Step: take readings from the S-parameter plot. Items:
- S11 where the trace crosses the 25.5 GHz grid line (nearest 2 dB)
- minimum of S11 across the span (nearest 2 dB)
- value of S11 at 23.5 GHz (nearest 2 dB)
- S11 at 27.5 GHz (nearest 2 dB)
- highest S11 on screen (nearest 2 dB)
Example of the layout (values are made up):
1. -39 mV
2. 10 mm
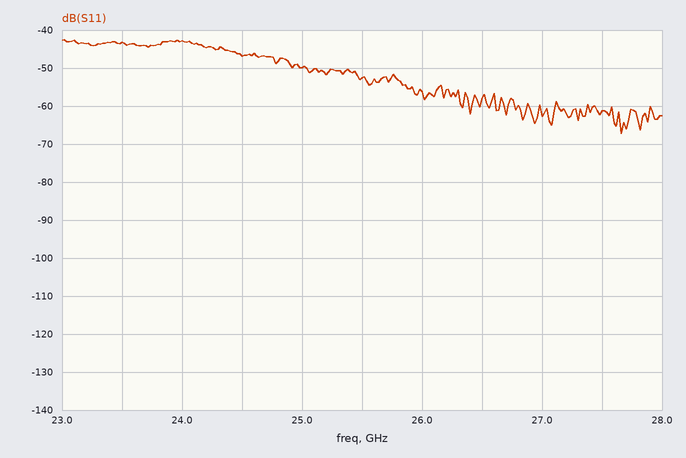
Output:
1. -52 dB
2. -68 dB
3. -44 dB
4. -62 dB
5. -42 dB
